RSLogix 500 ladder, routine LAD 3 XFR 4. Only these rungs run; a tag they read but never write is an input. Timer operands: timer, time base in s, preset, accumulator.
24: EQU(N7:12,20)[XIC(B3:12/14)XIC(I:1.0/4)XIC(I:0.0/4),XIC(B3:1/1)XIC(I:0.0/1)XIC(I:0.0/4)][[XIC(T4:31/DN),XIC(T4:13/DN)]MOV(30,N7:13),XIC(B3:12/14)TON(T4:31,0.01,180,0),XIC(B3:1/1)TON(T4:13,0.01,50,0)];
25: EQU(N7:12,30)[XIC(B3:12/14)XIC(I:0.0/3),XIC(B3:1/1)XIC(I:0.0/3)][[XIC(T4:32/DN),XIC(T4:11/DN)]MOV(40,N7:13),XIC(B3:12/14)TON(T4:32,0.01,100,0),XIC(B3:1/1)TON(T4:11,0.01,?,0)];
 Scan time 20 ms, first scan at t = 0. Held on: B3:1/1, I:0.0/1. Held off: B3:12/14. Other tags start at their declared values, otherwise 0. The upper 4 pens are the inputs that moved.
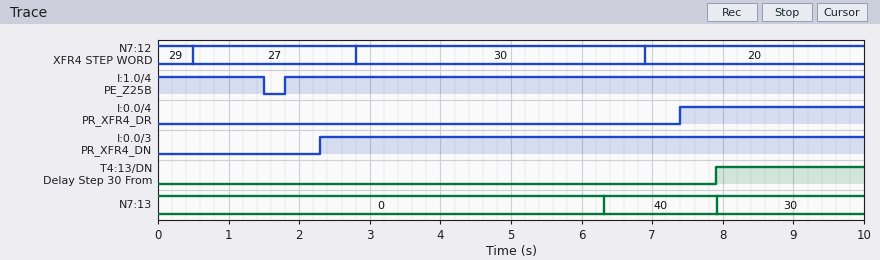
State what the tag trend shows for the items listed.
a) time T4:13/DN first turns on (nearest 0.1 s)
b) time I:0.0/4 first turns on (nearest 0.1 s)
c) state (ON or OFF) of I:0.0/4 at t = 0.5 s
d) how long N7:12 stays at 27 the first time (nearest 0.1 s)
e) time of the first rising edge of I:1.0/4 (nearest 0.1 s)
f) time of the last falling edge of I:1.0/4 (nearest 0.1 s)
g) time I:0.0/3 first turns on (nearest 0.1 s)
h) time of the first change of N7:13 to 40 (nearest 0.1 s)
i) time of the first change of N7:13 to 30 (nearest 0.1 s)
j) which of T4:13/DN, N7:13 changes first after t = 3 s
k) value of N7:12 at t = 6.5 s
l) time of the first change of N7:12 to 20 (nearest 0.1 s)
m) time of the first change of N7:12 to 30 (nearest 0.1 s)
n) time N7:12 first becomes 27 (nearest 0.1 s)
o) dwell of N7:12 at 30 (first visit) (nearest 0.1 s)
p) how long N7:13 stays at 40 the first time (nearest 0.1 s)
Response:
7.9 s
7.4 s
OFF
2.3 s
1.8 s
1.5 s
2.3 s
6.3 s
7.9 s
N7:13
30
6.9 s
2.8 s
0.5 s
4.1 s
1.6 s
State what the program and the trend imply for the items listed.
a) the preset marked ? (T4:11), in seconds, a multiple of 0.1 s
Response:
3.5 s
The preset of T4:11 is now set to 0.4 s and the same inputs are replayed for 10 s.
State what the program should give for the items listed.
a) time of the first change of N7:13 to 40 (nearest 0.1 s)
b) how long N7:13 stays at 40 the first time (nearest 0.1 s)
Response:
3.2 s
4.7 s
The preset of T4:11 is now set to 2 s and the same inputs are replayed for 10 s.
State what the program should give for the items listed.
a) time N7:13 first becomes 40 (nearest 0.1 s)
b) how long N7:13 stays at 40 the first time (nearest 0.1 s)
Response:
4.8 s
3.1 s
